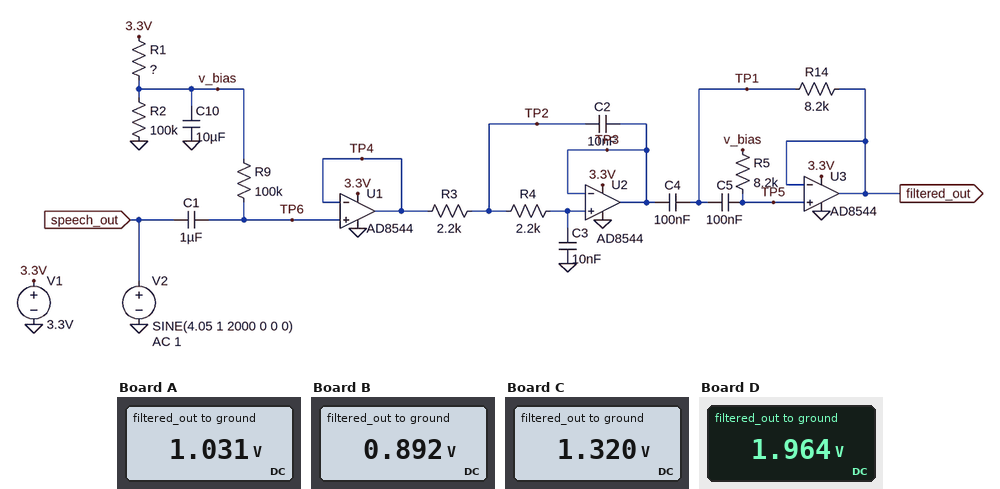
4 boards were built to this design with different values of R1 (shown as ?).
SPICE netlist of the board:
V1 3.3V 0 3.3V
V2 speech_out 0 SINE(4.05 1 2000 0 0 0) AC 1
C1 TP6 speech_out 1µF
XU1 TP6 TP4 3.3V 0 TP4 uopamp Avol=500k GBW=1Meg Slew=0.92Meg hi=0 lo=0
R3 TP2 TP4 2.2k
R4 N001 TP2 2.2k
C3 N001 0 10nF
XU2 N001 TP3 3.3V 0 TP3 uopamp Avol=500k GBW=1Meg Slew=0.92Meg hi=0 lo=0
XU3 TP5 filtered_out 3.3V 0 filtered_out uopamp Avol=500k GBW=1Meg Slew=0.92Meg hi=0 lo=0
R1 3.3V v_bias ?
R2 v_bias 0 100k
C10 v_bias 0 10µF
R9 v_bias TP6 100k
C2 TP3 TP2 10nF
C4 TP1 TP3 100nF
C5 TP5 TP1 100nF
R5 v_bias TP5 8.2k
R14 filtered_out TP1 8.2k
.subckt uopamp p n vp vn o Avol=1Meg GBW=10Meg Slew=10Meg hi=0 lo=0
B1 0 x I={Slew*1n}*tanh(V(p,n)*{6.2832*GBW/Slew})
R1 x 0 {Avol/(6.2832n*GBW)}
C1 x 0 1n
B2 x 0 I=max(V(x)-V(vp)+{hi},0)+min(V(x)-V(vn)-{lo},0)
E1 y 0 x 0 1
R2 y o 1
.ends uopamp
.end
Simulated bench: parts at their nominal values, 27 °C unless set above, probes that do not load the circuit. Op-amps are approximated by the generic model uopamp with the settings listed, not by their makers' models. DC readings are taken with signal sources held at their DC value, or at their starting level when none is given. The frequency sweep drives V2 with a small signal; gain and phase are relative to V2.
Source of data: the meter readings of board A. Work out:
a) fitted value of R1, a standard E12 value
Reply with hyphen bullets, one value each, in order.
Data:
- 220 kΩ
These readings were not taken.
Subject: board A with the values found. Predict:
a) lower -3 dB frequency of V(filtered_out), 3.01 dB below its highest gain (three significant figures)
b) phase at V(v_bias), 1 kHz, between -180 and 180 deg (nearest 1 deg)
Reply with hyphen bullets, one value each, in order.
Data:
- 280 Hz
- -84 deg
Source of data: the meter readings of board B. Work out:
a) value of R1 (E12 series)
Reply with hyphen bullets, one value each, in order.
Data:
- 270 kΩ
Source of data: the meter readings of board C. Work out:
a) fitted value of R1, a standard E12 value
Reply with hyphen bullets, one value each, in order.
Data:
- 150 kΩ
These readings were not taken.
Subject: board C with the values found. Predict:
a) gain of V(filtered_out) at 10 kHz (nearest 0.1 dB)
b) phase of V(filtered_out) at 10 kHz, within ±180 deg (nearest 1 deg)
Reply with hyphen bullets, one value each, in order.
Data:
- -9.3 dB
- -108 deg
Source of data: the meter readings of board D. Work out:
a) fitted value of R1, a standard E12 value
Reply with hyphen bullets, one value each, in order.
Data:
- 68 kΩ
